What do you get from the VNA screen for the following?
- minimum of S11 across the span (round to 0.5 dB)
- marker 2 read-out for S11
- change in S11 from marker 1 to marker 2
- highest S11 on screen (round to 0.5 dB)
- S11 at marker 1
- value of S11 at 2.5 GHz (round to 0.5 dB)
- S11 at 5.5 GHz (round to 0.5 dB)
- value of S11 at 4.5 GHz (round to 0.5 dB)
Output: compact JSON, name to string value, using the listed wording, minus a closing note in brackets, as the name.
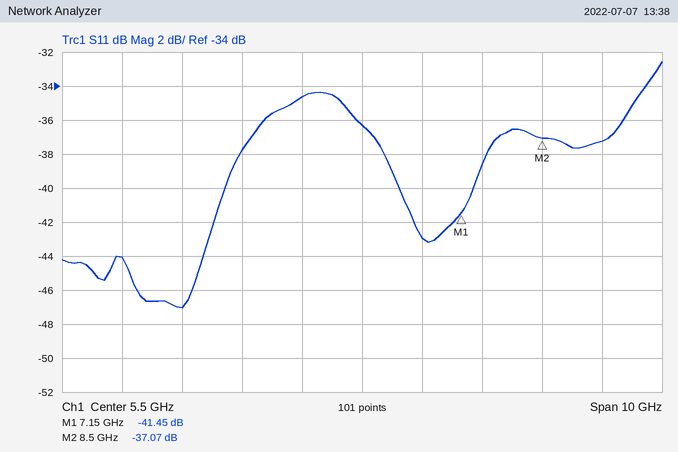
{"minimum of S11 across the span": "-47.0 dB", "marker 2 read-out for S11": "-37.07 dB", "change in S11 from marker 1 to marker 2": "4.38 dB", "highest S11 on screen": "-32.5 dB", "S11 at marker 1": "-41.45 dB", "value of S11 at 2.5 GHz": "-47.0 dB", "S11 at 5.5 GHz": "-36.5 dB", "value of S11 at 4.5 GHz": "-34.5 dB"}
